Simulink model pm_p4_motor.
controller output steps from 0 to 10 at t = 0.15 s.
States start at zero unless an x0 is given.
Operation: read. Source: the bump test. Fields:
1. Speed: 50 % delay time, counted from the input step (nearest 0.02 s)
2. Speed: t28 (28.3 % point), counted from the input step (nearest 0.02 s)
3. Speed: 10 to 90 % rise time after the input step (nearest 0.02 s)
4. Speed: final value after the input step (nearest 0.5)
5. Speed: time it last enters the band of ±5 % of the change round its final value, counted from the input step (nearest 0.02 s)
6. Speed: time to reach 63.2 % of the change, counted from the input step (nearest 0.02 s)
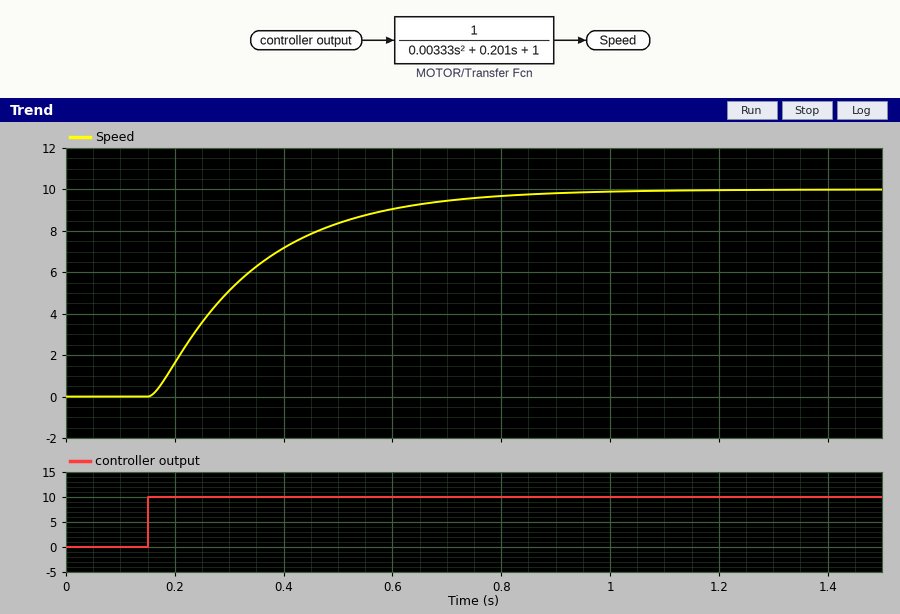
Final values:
0.14 s
0.08 s
0.40 s
10.0
0.56 s
0.20 s
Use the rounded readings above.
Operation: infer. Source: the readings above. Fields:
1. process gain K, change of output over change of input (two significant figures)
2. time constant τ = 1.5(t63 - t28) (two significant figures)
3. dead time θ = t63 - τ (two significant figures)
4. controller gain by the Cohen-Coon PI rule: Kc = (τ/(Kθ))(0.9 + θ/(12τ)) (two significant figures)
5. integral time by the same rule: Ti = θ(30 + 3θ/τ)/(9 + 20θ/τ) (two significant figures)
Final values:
1.0
0.18 s
0.020 s
8.2
0.054 s
